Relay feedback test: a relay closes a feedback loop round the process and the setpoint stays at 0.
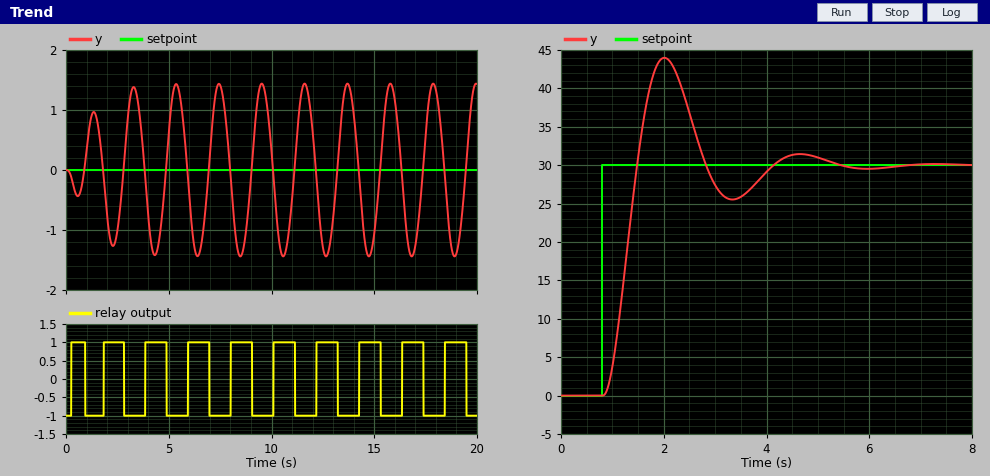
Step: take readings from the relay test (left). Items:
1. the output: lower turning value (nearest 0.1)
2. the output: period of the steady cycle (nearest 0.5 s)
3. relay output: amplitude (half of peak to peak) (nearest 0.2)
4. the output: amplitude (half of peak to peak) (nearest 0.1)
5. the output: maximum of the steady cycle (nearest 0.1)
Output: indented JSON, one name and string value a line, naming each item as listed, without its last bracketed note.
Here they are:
{
  "the output: lower turning value": "-1.4",
  "the output: period of the steady cycle": "2.0 s",
  "relay output: amplitude (half of peak to peak)": "1.0",
  "the output: amplitude (half of peak to peak)": "1.4",
  "the output: maximum of the steady cycle": "1.4"
}
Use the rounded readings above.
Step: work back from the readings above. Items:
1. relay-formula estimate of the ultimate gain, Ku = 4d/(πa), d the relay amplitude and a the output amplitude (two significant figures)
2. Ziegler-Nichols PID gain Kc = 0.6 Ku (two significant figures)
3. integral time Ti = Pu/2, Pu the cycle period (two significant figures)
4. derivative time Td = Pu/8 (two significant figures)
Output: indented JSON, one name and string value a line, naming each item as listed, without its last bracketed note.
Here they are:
{
  "relay-formula estimate of the ultimate gain, Ku = 4d/(πa), d the relay amplitude and a the output amplitude": "0.91",
  "Ziegler-Nichols PID gain Kc = 0.6 Ku": "0.55",
  "integral time Ti = Pu/2, Pu the cycle period": "1.0 s",
  "derivative time Td = Pu/8": "0.25 s"
}
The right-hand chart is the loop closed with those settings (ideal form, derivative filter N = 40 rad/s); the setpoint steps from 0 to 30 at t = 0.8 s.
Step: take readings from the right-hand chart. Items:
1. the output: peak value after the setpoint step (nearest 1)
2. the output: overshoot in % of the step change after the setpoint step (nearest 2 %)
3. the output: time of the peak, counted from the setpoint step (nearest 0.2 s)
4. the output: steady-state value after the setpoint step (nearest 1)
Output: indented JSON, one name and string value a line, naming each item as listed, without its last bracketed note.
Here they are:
{
  "the output: peak value after the setpoint step": "44",
  "the output: overshoot in % of the step change after the setpoint step": "46 %",
  "the output: time of the peak, counted from the setpoint step": "1.2 s",
  "the output: steady-state value after the setpoint step": "30"
}
